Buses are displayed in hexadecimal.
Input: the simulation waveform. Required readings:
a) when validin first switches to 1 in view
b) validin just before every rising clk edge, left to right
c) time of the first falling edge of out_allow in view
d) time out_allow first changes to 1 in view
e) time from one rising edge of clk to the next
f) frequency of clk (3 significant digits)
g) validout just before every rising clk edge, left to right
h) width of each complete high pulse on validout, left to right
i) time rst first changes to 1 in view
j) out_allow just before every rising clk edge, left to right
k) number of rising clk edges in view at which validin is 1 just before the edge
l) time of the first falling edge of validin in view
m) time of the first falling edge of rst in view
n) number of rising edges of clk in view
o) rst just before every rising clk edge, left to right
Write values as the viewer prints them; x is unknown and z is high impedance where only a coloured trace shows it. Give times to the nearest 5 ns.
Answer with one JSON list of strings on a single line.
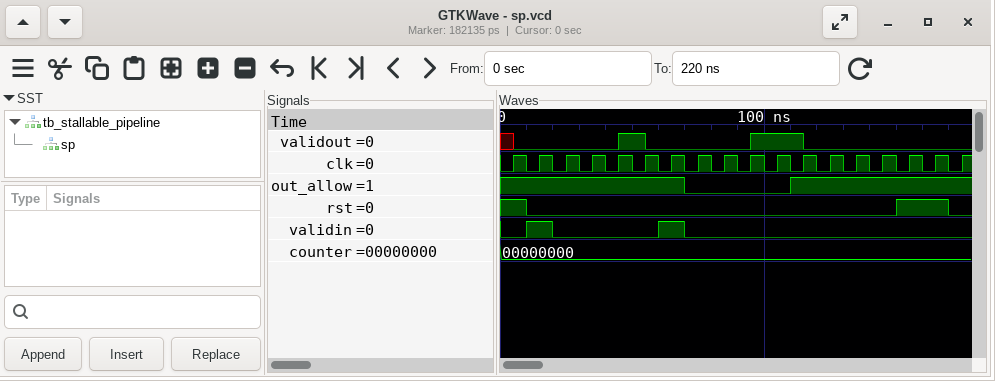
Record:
["10 ns", "0 1 0 0 0 0 1 0 0 0 0 0 0 0 0 0 0 0", "70 ns", "110 ns", "10 ns", "100 MHz", "x 0 0 0 0 1 0 0 0 0 1 1 0 0 0 0 0 0", "10 ns, 20 ns", "150 ns", "1 1 1 1 1 1 1 0 0 0 0 1 1 1 1 1 1 1", "2", "20 ns", "10 ns", "18", "1 0 0 0 0 0 0 0 0 0 0 0 0 0 0 1 1 0"]
